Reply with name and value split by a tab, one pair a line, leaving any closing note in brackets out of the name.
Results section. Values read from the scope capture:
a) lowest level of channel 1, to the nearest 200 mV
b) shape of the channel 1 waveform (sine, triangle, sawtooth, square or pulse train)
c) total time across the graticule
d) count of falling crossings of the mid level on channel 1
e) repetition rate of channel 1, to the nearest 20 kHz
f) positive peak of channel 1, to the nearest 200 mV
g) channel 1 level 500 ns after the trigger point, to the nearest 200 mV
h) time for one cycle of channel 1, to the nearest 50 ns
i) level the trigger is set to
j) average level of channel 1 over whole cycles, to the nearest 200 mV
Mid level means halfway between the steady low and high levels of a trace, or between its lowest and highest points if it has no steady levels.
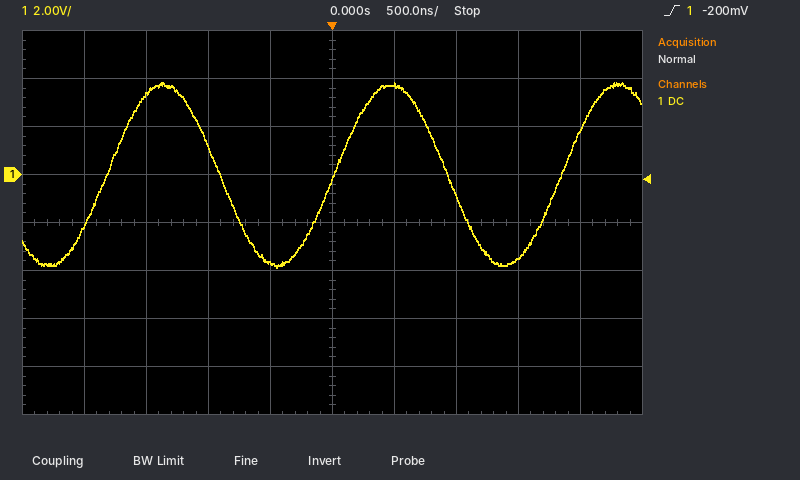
lowest level of channel 1, to the nearest 200 mV	-3.8 V
shape of the channel 1 waveform	sine
total time across the graticule	5 µs
count of falling crossings of the mid level on channel 1	2
repetition rate of channel 1, to the nearest 20 kHz	540 kHz
positive peak of channel 1, to the nearest 200 mV	3.8 V
channel 1 level 500 ns after the trigger point, to the nearest 200 mV	3.8 V
time for one cycle of channel 1, to the nearest 50 ns	1.85 µs
level the trigger is set to	-200 mV
average level of channel 1 over whole cycles, to the nearest 200 mV	0.0 V
